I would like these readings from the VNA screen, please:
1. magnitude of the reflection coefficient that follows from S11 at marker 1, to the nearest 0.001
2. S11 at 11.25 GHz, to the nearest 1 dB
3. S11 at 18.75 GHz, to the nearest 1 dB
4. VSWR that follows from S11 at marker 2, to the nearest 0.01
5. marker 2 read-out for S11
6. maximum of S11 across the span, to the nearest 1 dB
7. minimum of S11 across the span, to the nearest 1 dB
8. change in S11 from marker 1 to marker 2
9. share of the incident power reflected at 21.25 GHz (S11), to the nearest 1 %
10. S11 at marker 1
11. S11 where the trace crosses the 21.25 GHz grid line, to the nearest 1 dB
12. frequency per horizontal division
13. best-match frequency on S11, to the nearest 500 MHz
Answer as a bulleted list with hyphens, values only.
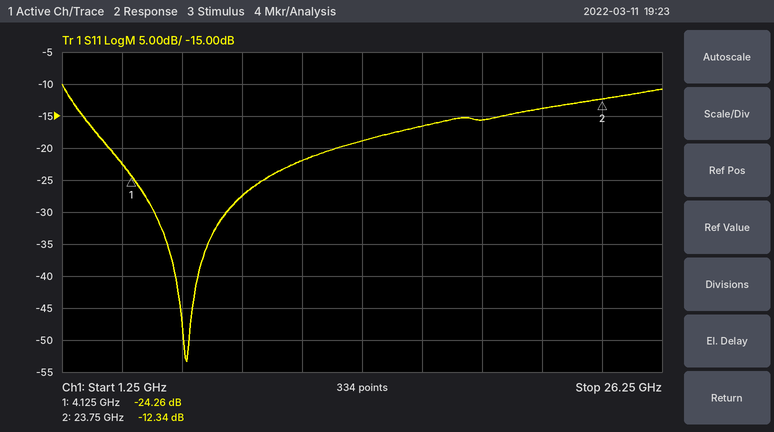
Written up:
- 0.061
- -22 dB
- -16 dB
- 1.64
- -12.34 dB
- -10 dB
- -53 dB
- 11.92 dB
- 4 %
- -24.26 dB
- -14 dB
- 2.5 GHz
- 6.5 GHz
